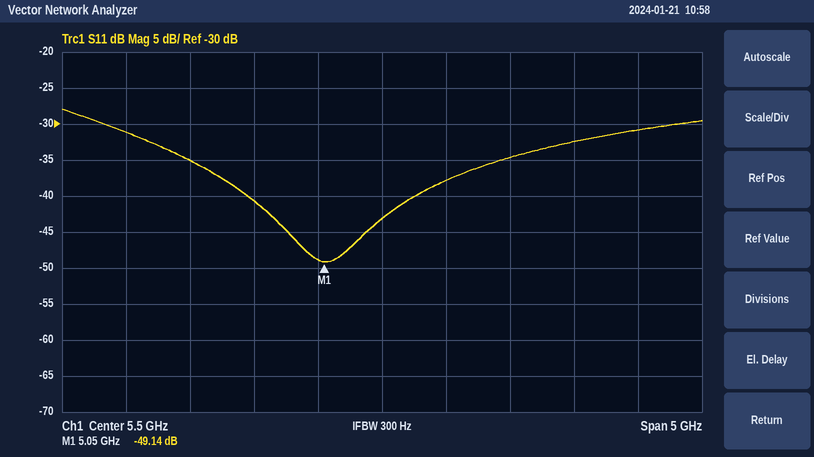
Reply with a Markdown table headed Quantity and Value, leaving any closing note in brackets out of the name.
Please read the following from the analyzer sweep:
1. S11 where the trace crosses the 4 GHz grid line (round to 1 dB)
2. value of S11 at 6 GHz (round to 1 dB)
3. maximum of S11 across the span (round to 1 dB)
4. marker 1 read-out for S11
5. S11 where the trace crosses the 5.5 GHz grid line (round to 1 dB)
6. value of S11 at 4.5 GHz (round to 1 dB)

| Quantity | Value |
|---|---|
| S11 where the trace crosses the 4 GHz grid line | -35 dB |
| value of S11 at 6 GHz | -38 dB |
| maximum of S11 across the span | -28 dB |
| marker 1 read-out for S11 | -49.14 dB |
| S11 where the trace crosses the 5.5 GHz grid line | -43 dB |
| value of S11 at 4.5 GHz | -41 dB |
